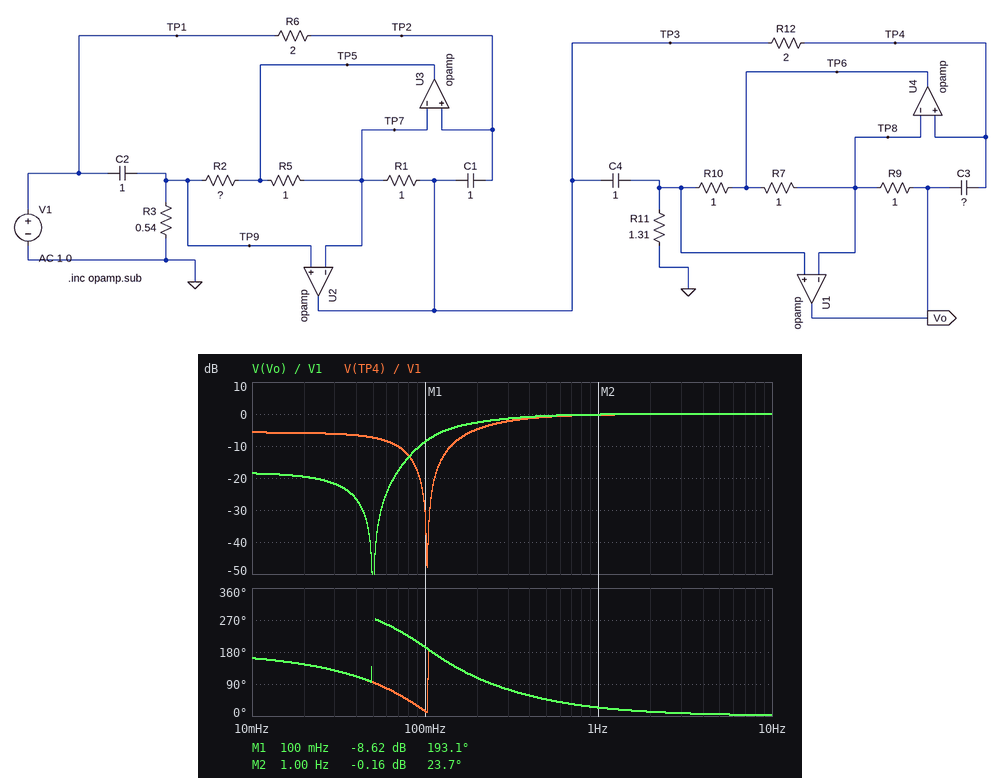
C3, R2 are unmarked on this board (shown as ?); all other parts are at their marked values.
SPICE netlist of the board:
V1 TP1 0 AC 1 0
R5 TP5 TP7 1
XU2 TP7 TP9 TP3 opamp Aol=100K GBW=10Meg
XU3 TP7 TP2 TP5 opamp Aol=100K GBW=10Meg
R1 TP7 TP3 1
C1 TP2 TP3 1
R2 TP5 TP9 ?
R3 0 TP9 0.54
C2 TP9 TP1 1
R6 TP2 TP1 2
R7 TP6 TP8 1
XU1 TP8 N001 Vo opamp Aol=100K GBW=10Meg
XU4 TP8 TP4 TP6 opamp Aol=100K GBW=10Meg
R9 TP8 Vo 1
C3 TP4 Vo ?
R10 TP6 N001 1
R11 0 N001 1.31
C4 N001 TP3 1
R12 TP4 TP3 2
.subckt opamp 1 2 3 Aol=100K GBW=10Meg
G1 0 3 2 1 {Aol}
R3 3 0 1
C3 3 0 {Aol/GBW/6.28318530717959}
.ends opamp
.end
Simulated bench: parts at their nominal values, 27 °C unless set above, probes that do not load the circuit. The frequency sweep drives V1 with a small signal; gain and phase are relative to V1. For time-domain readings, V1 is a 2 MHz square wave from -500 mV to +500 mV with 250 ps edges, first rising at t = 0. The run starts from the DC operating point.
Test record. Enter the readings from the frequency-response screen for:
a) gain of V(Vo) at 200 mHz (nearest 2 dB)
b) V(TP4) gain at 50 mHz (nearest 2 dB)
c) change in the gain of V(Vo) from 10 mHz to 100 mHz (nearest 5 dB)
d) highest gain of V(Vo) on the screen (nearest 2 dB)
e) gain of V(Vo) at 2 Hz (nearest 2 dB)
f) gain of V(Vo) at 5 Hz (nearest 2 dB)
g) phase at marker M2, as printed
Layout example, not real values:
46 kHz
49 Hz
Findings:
-2 dB
-8 dB
10 dB
0 dB
0 dB
0 dB
23.7 deg
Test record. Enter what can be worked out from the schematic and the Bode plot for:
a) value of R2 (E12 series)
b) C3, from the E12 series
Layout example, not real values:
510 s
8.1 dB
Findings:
0.82 Ω
1.2 F
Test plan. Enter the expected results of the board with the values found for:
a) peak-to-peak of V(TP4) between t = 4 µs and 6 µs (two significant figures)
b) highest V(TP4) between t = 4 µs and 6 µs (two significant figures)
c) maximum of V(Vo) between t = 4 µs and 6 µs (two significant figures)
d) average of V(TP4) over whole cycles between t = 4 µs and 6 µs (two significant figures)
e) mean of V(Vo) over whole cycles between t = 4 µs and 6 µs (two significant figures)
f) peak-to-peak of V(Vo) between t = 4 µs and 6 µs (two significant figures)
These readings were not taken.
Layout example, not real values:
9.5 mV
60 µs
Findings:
1.8 V
1.7 V
1.5 V
760 mV
560 mV
1.8 V
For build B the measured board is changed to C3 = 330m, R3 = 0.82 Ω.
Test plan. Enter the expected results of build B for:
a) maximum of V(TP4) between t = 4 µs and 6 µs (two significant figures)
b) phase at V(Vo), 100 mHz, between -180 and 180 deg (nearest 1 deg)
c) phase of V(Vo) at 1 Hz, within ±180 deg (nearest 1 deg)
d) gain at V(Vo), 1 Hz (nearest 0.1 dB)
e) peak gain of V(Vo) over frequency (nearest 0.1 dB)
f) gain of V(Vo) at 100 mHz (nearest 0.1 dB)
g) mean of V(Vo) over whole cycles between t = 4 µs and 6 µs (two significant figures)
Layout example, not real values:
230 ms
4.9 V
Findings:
1.4 V
-98 deg
18 deg
0.2 dB
2.1 dB
-36.6 dB
500 mV
